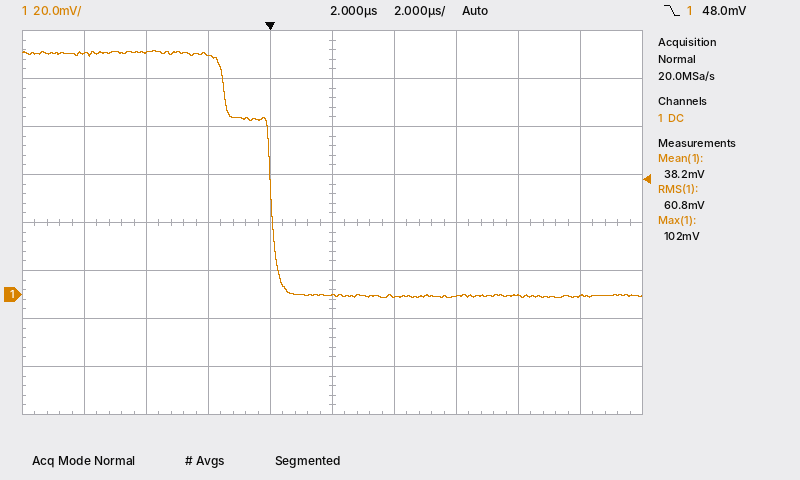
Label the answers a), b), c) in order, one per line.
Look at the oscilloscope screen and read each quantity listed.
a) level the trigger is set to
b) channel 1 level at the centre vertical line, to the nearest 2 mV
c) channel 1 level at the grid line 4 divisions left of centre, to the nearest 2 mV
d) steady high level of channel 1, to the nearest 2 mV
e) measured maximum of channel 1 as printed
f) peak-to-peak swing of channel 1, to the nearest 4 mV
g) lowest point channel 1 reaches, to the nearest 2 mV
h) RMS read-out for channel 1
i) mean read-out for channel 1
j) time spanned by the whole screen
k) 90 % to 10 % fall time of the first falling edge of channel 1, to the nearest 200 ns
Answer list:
a) 48.0 mV
b) 0 mV
c) 100 mV
d) 100 mV
e) 102 mV
f) 104 mV
g) -2 mV
h) 60.8 mV
i) 38.2 mV
j) 20 µs
k) 1.8 µs
